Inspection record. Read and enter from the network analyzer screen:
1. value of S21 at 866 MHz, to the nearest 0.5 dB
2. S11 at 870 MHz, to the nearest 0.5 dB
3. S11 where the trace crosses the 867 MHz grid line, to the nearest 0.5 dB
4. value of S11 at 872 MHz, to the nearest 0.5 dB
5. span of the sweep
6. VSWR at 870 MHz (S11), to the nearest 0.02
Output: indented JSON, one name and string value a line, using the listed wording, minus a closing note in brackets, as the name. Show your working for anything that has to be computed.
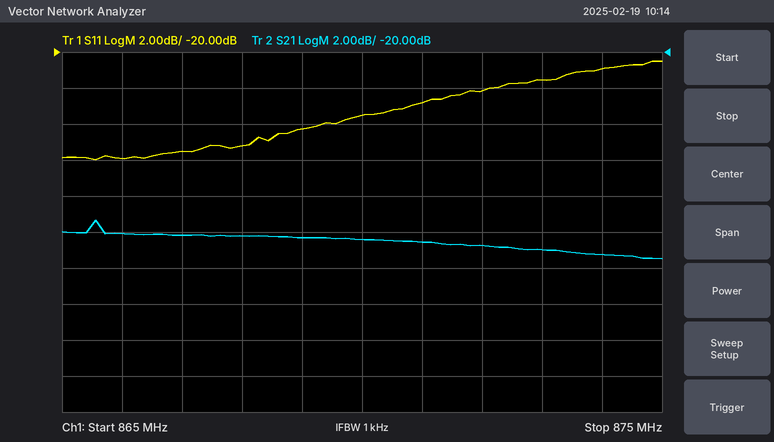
{
  "value of S21 at 866 MHz, to the nearest 0.5 dB": "-30.0 dB",
  "S11 at 870 MHz, to the nearest 0.5 dB": "-23.5 dB",
  "S11 where the trace crosses the 867 MHz grid line, to the nearest 0.5 dB": "-25.5 dB",
  "value of S11 at 872 MHz, to the nearest 0.5 dB": "-22.0 dB",
  "span of the sweep": "10 MHz",
  "VSWR at 870 MHz (S11), to the nearest 0.02": "|Γ| = 10^(-23.5/20) = 0.0668; VSWR = (1 + 0.0668)/(1 − 0.0668) ≈ 1.14"
}
